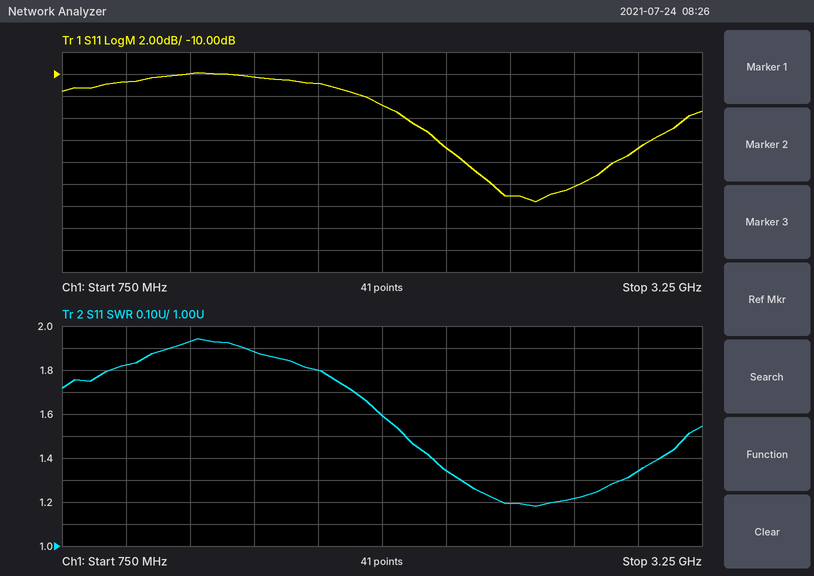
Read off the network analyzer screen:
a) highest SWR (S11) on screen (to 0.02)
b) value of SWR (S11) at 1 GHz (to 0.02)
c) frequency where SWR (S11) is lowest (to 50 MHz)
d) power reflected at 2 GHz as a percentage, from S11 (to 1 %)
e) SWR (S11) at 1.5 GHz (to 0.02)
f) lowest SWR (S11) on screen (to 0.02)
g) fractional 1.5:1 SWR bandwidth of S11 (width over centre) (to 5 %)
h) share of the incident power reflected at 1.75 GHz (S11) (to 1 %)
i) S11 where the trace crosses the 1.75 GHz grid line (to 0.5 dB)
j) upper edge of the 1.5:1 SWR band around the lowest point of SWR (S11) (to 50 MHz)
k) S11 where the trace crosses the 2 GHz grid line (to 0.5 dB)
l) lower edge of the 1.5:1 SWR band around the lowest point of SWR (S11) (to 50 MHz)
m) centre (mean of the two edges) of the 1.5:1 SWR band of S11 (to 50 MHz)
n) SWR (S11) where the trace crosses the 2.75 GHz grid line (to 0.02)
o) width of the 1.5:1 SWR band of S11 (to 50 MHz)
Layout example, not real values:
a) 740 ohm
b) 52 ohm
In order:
a) 1.94
b) 1.82
c) 2.60 GHz
d) 5 %
e) 1.88
f) 1.18
g) 40 %
h) 8 %
i) -11.0 dB
j) 3.20 GHz
k) -13.0 dB
l) 2.10 GHz
m) 2.65 GHz
n) 1.22
o) 1.10 GHz
